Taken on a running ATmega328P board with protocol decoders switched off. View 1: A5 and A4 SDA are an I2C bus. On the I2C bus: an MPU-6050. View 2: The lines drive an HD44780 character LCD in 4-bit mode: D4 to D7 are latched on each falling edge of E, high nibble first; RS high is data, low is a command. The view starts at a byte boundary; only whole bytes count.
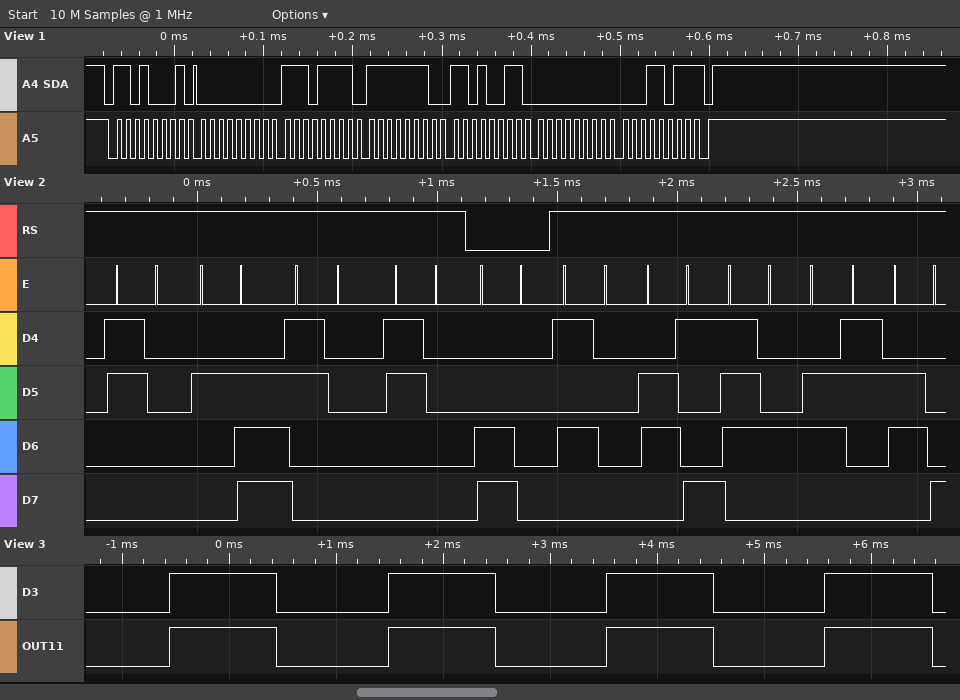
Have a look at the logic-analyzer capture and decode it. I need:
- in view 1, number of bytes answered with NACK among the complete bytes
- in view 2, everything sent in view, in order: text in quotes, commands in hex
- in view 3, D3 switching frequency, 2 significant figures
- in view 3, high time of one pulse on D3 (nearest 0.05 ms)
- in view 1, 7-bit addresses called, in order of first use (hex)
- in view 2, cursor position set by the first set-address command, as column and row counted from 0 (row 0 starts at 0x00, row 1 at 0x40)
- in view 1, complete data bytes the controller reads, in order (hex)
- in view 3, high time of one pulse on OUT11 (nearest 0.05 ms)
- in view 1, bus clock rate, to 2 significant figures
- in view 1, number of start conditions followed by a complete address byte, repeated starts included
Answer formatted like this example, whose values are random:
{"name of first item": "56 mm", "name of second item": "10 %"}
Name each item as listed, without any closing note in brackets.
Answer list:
{"in view 1, number of bytes answered with NACK among the complete bytes": "1", "in view 2, everything sent in view, in order: text in quotes, commands in hex": "\"0.00\" 0xC0 \"Pitch\"", "in view 3, D3 switching frequency, 2 significant figures": "490 Hz", "in view 3, high time of one pulse on D3": "1.00 ms", "in view 1, 7-bit addresses called, in order of first use": "0x68", "in view 2, cursor position set by the first set-address command, as column and row counted from 0": "column 0, row 1", "in view 1, complete data bytes the controller reads, in order": "00 EF FE D3 00 1B", "in view 3, high time of one pulse on OUT11": "1.00 ms", "in view 1, bus clock rate, to 2 significant figures": "100 kHz", "in view 1, number of start conditions followed by a complete address byte, repeated starts included": "1"}
